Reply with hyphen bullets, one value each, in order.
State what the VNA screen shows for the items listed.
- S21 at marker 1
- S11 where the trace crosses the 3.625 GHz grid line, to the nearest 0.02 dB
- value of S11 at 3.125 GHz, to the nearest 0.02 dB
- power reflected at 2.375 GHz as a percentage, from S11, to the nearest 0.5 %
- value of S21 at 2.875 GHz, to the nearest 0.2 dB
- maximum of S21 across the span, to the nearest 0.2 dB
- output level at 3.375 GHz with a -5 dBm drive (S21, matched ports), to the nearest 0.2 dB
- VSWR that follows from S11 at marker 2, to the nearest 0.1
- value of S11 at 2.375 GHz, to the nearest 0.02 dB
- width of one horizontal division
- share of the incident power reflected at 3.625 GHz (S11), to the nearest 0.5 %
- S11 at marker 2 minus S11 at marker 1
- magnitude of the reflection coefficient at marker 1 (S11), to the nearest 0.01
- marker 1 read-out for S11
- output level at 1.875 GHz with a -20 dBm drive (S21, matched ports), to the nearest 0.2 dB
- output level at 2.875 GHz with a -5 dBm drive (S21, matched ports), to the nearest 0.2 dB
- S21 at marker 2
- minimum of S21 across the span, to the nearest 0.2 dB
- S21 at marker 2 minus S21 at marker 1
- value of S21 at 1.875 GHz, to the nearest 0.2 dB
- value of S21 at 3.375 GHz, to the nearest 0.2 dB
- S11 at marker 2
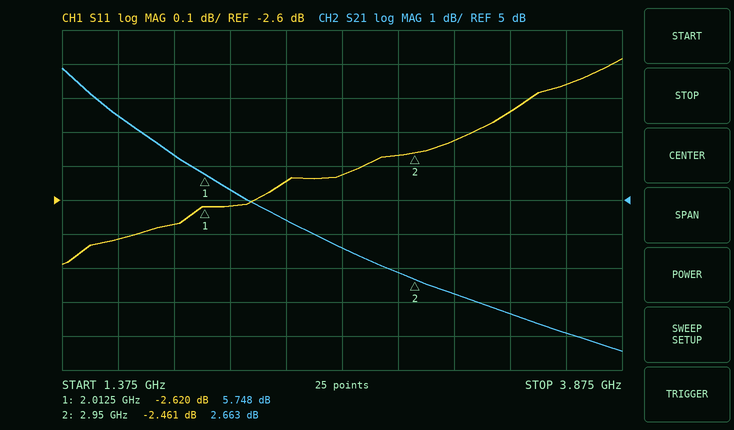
- 5.748 dB
- -2.26 dB
- -2.42 dB
- 55.5 %
- 2.8 dB
- 8.8 dB
- -3.4 dBm
- 7.1
- -2.54 dB
- 250 MHz
- 59.5 %
- 0.159 dB
- 0.74
- -2.620 dB
- -13.6 dBm
- -2.2 dBm
- 2.663 dB
- 0.6 dB
- -3.085 dB
- 6.4 dB
- 1.6 dB
- -2.461 dB
